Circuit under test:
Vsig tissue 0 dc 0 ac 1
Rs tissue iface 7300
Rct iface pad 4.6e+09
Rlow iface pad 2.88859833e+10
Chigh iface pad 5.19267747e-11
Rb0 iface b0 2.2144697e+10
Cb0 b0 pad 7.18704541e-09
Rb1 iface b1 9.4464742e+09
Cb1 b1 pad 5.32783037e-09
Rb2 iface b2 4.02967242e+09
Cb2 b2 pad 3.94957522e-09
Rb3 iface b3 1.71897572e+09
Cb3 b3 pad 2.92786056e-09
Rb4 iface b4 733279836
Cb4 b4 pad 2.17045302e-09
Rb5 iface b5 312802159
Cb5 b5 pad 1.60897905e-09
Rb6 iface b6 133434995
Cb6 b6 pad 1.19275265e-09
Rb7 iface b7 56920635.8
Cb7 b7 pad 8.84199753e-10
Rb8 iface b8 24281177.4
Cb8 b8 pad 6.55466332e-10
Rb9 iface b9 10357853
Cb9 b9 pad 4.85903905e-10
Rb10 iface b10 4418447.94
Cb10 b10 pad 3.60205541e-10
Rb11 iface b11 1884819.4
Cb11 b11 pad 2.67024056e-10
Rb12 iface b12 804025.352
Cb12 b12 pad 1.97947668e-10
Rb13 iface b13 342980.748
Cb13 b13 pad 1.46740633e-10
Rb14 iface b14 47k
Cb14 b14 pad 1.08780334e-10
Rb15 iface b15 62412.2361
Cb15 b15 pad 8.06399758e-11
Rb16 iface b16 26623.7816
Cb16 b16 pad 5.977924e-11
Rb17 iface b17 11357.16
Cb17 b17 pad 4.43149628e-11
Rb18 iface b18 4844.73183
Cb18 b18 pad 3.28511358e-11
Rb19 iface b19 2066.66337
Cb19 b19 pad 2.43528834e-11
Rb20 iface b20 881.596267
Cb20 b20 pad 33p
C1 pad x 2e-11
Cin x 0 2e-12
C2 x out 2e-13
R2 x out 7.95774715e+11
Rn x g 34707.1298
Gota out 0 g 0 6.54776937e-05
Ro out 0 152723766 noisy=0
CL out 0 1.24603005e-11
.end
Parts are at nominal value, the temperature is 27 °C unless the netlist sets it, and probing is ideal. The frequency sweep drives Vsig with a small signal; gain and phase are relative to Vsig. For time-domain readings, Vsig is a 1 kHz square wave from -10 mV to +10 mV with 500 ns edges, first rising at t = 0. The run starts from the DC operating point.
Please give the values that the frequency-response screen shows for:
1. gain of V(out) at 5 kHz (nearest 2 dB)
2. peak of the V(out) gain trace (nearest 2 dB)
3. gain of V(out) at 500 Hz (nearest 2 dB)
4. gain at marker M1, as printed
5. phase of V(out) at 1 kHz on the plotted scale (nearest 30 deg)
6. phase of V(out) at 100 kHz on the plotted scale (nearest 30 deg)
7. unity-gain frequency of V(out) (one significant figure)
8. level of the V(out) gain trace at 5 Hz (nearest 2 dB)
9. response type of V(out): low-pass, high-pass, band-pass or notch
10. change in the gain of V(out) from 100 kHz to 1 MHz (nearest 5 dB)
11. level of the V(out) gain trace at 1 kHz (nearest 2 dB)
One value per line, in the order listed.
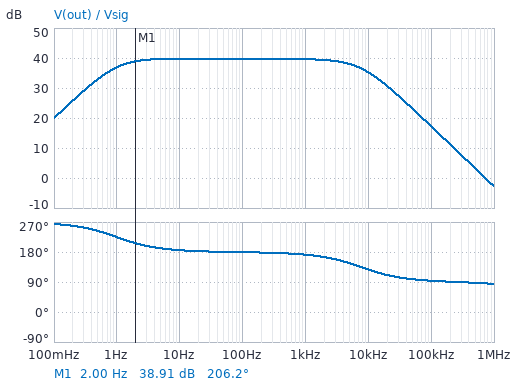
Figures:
38 dB
40 dB
40 dB
38.91 dB
180 deg
90 deg
700 kHz
40 dB
band-pass
-20 dB
40 dB
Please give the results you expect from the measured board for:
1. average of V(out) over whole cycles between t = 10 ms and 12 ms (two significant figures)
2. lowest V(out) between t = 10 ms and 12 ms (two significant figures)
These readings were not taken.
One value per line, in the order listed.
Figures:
-920 mV
-1.9 V
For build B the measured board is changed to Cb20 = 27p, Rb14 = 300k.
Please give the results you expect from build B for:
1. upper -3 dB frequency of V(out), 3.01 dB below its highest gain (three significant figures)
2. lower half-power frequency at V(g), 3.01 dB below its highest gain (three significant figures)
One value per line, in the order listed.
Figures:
7.11 kHz
7.77 kHz
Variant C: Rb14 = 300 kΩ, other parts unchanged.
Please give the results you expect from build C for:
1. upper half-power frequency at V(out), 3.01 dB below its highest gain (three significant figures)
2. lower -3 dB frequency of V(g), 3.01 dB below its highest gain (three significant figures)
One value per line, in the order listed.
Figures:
7.12 kHz
7.77 kHz
